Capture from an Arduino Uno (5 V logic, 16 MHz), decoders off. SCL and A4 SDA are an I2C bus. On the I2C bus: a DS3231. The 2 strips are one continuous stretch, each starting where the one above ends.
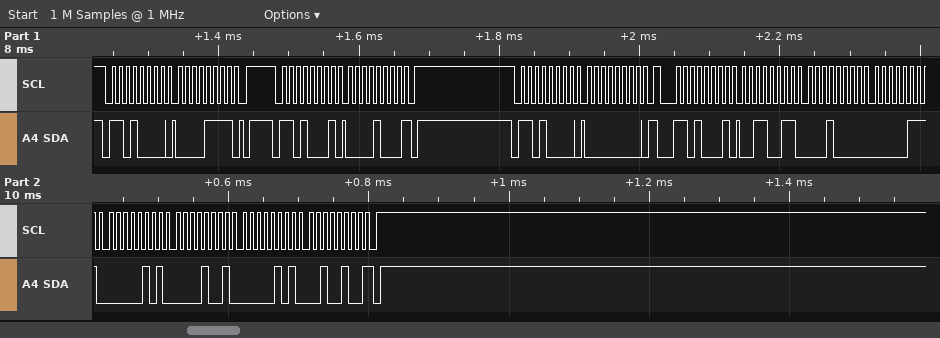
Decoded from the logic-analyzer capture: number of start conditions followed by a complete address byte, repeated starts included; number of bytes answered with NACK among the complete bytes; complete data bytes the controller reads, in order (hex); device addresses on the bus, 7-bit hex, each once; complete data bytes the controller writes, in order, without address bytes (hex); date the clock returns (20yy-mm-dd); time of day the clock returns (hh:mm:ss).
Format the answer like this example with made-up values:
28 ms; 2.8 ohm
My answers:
4; 2; 08 33 10 07 05 09 05 24; 0x68; 0F 00; 2024-05-09; 07:10:33
